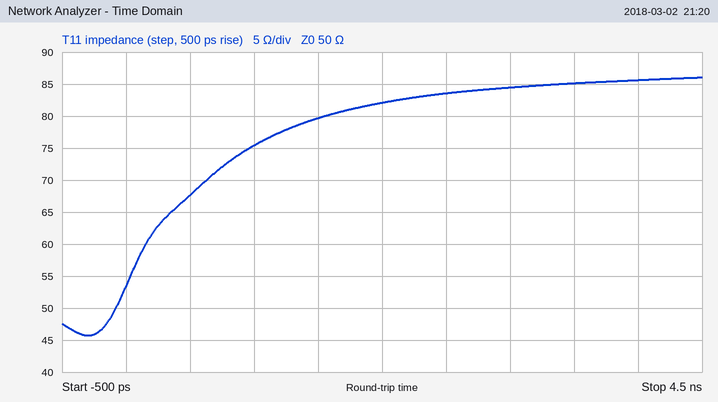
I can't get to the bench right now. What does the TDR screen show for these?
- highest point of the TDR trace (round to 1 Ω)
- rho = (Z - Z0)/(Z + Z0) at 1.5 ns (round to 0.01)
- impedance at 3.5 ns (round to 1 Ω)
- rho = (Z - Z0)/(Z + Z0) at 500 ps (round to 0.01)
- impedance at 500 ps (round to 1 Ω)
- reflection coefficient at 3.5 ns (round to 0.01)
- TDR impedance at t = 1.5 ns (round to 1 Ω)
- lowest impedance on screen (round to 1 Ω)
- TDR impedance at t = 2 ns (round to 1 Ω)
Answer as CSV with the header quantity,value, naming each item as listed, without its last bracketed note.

quantity,value
highest point of the TDR trace,86 Ω
rho = (Z - Z0)/(Z + Z0) at 1.5 ns,+0.23
impedance at 3.5 ns,85 Ω
rho = (Z - Z0)/(Z + Z0) at 500 ps,+0.15
impedance at 500 ps,68 Ω
reflection coefficient at 3.5 ns,+0.26
TDR impedance at t = 1.5 ns,80 Ω
lowest impedance on screen,46 Ω
TDR impedance at t = 2 ns,82 Ω
